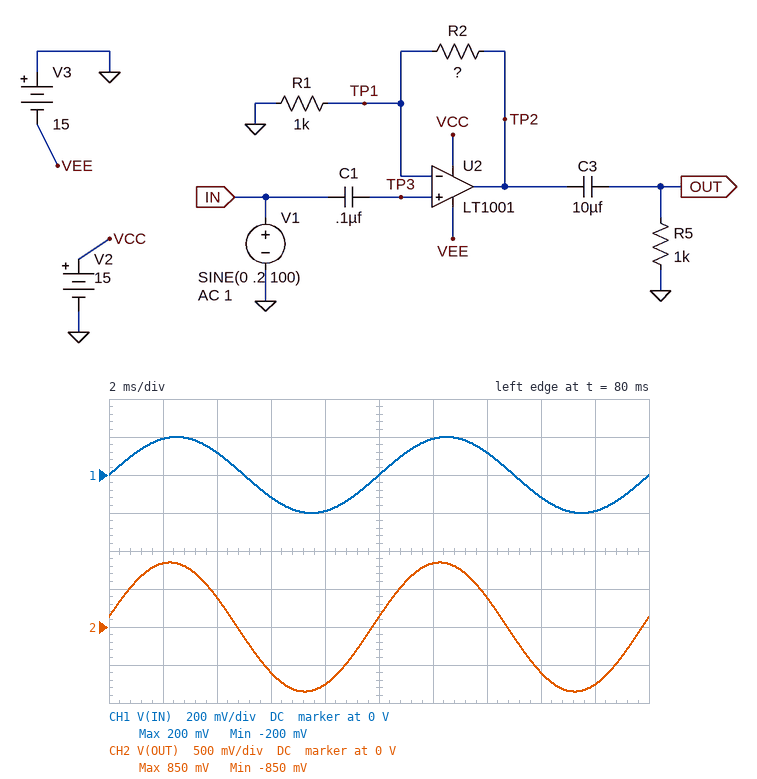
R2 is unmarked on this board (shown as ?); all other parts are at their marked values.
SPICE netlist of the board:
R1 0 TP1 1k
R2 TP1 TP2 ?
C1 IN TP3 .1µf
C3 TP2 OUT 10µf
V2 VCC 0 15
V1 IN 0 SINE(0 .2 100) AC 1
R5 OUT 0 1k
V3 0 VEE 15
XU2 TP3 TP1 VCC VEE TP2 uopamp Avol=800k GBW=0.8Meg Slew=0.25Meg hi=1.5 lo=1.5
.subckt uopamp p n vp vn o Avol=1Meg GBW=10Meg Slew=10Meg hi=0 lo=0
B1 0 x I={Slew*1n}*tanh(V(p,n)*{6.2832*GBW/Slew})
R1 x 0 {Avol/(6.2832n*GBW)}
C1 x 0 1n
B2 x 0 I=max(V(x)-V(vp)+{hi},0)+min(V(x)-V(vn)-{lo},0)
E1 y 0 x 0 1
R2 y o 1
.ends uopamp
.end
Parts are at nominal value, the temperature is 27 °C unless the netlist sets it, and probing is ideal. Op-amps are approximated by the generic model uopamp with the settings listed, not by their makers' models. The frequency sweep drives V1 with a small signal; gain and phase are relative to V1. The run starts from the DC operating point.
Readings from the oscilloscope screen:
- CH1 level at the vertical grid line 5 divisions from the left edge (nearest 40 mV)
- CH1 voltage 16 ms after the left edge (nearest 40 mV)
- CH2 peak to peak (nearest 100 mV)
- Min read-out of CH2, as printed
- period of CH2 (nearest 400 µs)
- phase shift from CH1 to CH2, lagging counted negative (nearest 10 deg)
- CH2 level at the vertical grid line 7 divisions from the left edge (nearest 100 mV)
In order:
0 V
-120 mV
1.7 V
-850 mV
10.0 ms
10 deg
400 mV
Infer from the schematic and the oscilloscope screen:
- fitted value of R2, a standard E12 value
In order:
3.3 kΩ
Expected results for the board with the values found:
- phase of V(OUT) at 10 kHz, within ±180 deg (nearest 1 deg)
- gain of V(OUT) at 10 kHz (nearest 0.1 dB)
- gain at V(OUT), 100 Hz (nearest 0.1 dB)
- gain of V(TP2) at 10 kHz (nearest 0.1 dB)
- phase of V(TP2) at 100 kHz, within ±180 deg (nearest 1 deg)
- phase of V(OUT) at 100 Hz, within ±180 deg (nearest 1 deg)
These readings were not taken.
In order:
-3 deg
12.7 dB
12.6 dB
12.7 dB
-28 deg
9 deg
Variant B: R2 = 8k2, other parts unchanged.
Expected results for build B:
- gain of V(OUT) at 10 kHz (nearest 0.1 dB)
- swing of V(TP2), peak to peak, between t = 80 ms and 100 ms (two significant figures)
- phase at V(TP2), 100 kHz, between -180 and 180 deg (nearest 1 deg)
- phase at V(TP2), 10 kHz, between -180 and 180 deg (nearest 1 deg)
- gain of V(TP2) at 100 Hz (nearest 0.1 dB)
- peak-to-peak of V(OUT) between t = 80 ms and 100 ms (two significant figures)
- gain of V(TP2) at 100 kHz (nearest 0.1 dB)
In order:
19.2 dB
3.7 V
-49 deg
-7 deg
19.3 dB
3.6 V
15.6 dB
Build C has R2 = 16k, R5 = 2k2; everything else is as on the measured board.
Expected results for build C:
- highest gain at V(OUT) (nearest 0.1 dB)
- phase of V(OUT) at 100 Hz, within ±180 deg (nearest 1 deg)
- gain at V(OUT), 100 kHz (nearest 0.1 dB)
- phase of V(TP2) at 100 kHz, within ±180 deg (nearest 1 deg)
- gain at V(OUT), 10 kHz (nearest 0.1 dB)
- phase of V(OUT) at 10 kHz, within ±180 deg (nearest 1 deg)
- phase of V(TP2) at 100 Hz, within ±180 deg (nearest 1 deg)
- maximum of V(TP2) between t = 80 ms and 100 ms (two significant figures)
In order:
24.6 dB
4 deg
17.2 dB
-65 deg
24.4 dB
-12 deg
0 deg
3.4 V
